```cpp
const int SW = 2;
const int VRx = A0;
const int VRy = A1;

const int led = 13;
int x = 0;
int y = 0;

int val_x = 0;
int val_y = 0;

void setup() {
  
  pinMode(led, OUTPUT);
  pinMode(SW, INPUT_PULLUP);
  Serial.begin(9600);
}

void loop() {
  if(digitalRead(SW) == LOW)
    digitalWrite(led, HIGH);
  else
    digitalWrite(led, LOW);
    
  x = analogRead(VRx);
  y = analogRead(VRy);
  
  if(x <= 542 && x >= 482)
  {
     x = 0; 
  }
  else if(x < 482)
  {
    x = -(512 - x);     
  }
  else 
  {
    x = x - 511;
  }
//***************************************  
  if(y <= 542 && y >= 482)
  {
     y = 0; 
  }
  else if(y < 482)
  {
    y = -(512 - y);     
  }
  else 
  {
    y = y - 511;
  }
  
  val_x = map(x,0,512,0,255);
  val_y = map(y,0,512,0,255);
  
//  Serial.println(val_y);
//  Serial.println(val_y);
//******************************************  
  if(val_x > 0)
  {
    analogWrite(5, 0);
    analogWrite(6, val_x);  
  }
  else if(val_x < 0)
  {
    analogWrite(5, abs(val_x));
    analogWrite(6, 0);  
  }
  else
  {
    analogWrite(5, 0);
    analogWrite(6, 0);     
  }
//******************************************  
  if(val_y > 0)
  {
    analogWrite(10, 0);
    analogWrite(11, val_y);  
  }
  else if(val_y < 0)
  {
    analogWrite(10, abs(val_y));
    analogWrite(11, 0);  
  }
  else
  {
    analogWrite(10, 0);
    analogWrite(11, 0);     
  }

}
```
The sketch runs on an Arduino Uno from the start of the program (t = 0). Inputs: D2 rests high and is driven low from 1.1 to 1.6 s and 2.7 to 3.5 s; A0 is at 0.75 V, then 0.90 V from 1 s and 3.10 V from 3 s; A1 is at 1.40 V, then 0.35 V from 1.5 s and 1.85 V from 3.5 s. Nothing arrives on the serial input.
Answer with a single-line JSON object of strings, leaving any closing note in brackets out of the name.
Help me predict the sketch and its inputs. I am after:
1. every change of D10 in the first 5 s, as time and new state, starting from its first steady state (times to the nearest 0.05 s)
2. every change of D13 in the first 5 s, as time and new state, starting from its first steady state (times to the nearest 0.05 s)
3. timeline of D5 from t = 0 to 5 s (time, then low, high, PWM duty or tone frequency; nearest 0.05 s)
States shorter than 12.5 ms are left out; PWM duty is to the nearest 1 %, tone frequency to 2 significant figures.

{"every change of D10 in the first 5 s, as time and new state, starting from its first steady state": "0 s PWM 44 %; 1.5 s PWM 86 %; 3.5 s PWM 26 %", "every change of D13 in the first 5 s, as time and new state, starting from its first steady state": "0 s low; 1.1 s high; 1.6 s low; 2.7 s high; 3.5 s low", "timeline of D5 from t = 0 to 5 s": "0 s PWM 70 %; 1 s PWM 64 %; 3 s low"}
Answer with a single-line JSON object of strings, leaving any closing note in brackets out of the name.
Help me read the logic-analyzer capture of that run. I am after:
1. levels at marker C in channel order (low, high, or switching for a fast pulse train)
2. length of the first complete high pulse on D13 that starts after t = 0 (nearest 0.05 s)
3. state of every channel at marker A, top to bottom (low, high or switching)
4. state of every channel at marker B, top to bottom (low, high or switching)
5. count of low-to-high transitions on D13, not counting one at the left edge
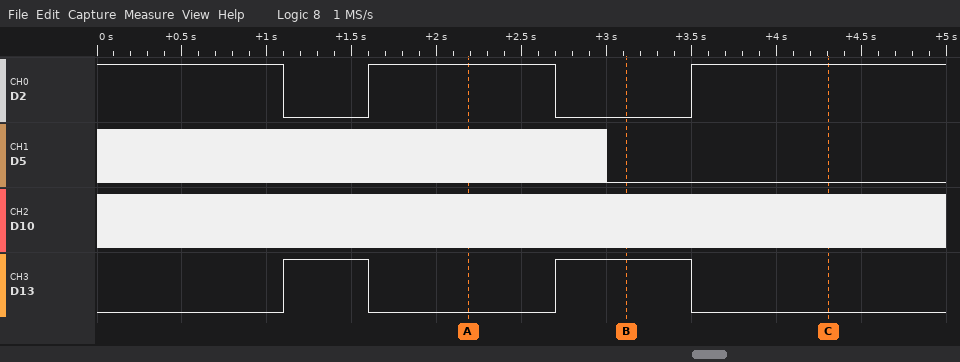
{"levels at marker C in channel order": "D2 high, D5 low, D10 switching, D13 low", "length of the first complete high pulse on D13 that starts after t = 0": "0.50 s", "state of every channel at marker A, top to bottom": "D2 high, D5 switching, D10 switching, D13 low", "state of every channel at marker B, top to bottom": "D2 low, D5 low, D10 switching, D13 high", "count of low-to-high transitions on D13, not counting one at the left edge": "2"}
